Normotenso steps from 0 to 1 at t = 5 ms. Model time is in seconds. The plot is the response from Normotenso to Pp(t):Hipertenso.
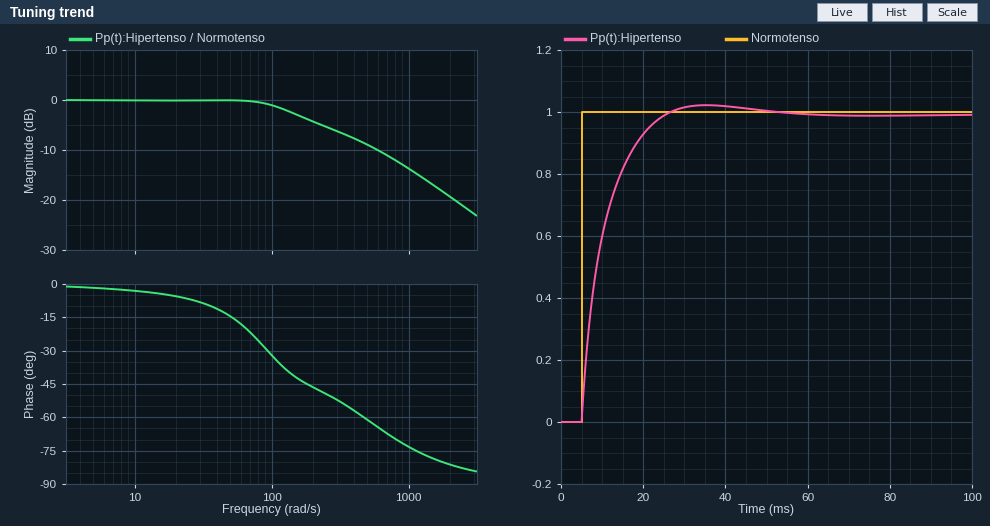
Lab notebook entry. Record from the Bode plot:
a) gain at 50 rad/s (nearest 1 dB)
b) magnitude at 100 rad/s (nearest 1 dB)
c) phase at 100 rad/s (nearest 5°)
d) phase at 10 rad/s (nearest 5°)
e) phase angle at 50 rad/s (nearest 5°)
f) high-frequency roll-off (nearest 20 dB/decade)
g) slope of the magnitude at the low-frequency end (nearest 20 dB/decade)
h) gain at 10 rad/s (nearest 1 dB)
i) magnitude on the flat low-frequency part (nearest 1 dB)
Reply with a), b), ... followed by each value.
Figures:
a) 0 dB
b) -1 dB
c) -30°
d) -5°
e) -15°
f) -20 dB/decade
g) 0 dB/decade
h) 0 dB
i) 0 dB
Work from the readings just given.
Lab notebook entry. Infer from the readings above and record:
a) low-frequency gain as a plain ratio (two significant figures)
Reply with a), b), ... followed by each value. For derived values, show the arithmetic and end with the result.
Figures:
a) 10^(0 / 20) = 1.0
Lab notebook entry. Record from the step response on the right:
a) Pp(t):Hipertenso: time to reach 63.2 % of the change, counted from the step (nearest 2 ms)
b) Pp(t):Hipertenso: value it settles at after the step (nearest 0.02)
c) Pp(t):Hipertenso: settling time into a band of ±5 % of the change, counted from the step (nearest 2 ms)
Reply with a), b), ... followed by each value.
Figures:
a) 6 ms
b) 1.00
c) 16 ms
